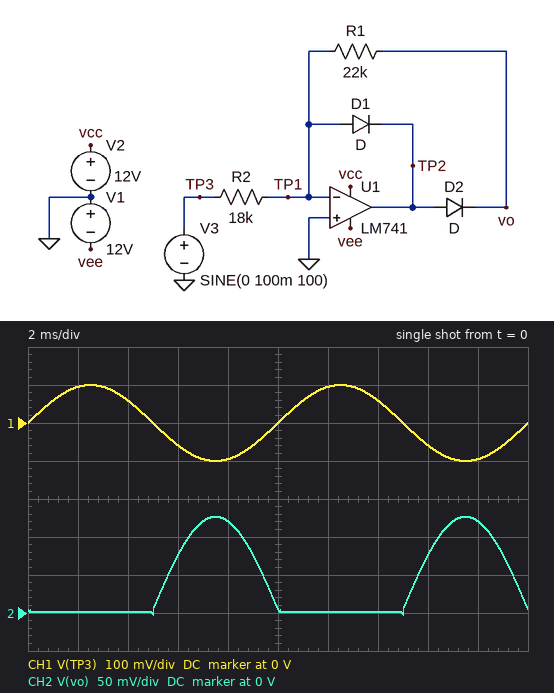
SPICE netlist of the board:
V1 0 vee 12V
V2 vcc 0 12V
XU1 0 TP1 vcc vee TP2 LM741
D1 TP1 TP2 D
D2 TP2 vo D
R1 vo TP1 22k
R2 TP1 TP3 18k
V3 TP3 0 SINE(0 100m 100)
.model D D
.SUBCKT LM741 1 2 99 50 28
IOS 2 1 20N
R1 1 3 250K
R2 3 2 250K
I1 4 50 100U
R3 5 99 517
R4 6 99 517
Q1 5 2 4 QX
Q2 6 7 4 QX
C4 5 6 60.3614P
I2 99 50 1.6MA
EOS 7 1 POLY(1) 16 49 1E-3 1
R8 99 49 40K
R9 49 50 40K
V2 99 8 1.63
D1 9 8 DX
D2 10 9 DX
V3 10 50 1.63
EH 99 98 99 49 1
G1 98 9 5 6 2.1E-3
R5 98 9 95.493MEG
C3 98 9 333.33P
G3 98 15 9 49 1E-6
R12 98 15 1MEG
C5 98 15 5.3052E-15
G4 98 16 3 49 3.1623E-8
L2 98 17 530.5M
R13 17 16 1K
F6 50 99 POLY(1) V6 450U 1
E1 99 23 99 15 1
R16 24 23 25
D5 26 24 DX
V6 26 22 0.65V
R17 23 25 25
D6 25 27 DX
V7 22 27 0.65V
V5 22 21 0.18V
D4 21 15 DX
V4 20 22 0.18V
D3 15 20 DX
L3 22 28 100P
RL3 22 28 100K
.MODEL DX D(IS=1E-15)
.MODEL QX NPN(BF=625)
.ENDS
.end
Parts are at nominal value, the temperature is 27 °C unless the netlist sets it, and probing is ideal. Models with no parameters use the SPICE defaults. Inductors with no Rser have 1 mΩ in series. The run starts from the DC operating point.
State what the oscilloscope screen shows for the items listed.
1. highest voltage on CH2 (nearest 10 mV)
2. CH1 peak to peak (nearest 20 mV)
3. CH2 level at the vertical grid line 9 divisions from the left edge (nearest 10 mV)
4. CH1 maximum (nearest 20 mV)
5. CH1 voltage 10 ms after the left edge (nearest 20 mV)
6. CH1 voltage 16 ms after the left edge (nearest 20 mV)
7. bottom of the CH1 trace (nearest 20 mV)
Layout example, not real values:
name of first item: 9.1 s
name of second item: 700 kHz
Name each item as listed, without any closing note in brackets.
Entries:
highest voltage on CH2: 130 mV
CH1 peak to peak: 200 mV
CH2 level at the vertical grid line 9 divisions from the left edge: 120 mV
CH1 maximum: 100 mV
CH1 voltage 10 ms after the left edge: 0 V
CH1 voltage 16 ms after the left edge: -60 mV
bottom of the CH1 trace: -100 mV
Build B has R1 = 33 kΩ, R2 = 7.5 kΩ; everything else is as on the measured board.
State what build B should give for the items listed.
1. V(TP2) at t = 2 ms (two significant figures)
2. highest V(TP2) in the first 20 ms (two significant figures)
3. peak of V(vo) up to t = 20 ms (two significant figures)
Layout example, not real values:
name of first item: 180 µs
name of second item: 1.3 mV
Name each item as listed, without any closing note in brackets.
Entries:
V(TP2) at t = 2 ms: -540 mV
highest V(TP2) in the first 20 ms: 990 mV
peak of V(vo) up to t = 20 ms: 450 mV
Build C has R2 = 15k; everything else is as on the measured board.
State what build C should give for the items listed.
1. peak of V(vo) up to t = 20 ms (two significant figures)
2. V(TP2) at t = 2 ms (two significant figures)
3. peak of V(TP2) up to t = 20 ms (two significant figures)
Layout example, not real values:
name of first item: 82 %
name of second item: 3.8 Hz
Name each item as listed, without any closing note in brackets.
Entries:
peak of V(vo) up to t = 20 ms: 150 mV
V(TP2) at t = 2 ms: -520 mV
peak of V(TP2) up to t = 20 ms: 680 mV
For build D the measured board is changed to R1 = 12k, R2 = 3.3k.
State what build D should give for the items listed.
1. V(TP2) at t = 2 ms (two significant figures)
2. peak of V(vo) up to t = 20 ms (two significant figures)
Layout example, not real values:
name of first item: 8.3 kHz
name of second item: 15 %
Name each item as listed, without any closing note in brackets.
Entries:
V(TP2) at t = 2 ms: -560 mV
peak of V(vo) up to t = 20 ms: 370 mV
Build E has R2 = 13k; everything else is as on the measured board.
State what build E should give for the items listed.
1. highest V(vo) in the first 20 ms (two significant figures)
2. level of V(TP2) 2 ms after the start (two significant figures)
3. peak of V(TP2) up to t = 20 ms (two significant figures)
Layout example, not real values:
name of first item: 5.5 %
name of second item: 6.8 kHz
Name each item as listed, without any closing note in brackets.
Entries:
highest V(vo) in the first 20 ms: 170 mV
level of V(TP2) 2 ms after the start: -530 mV
peak of V(TP2) up to t = 20 ms: 700 mV
